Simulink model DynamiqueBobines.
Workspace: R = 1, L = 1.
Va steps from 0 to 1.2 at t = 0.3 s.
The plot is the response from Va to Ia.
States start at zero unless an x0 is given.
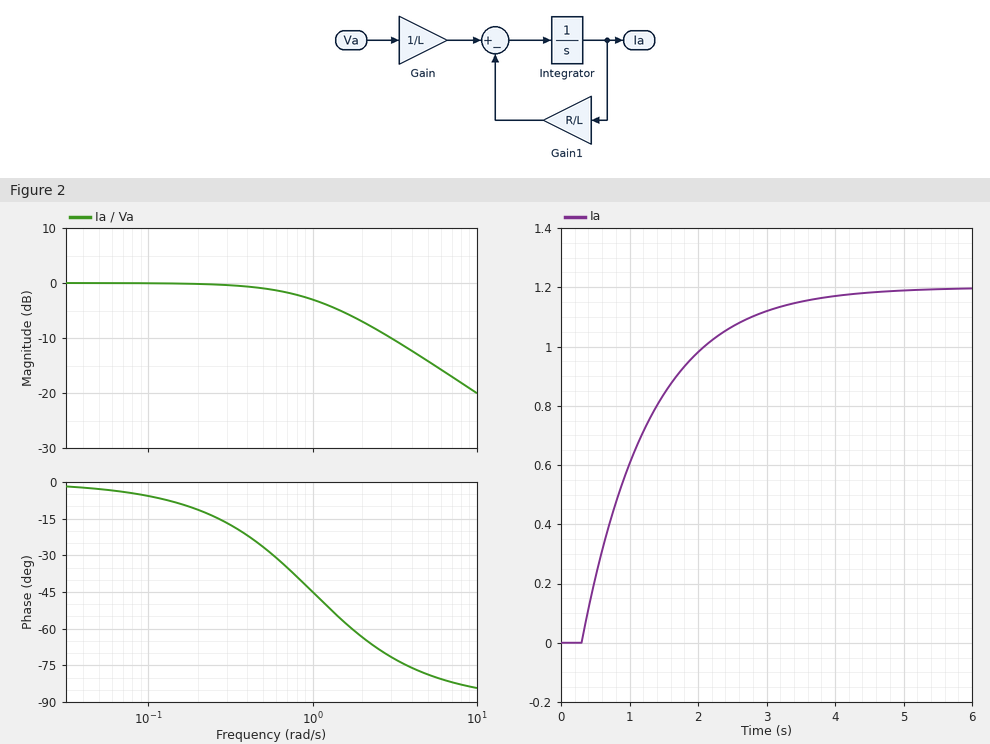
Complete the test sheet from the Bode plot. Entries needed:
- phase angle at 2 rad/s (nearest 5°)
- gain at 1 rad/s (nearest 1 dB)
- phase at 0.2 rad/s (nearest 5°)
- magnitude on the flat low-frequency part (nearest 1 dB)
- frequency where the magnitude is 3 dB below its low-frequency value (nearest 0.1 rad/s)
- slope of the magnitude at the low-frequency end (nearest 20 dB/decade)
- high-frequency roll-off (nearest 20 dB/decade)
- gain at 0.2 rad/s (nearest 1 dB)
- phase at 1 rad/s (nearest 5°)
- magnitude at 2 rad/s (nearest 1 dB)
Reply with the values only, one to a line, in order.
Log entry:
-65°
-3 dB
-10°
0 dB
1.0 rad/s
0 dB/decade
-20 dB/decade
0 dB
-45°
-7 dB
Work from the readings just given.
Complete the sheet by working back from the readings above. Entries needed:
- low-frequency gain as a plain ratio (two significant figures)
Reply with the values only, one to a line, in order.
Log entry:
1.0
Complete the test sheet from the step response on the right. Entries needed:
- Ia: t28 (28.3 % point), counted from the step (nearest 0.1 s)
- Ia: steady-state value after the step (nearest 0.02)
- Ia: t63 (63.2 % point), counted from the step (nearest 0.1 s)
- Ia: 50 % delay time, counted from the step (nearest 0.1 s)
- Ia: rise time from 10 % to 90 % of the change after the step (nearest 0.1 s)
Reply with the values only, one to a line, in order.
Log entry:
0.3 s
1.20
1.0 s
0.7 s
2.2 s
